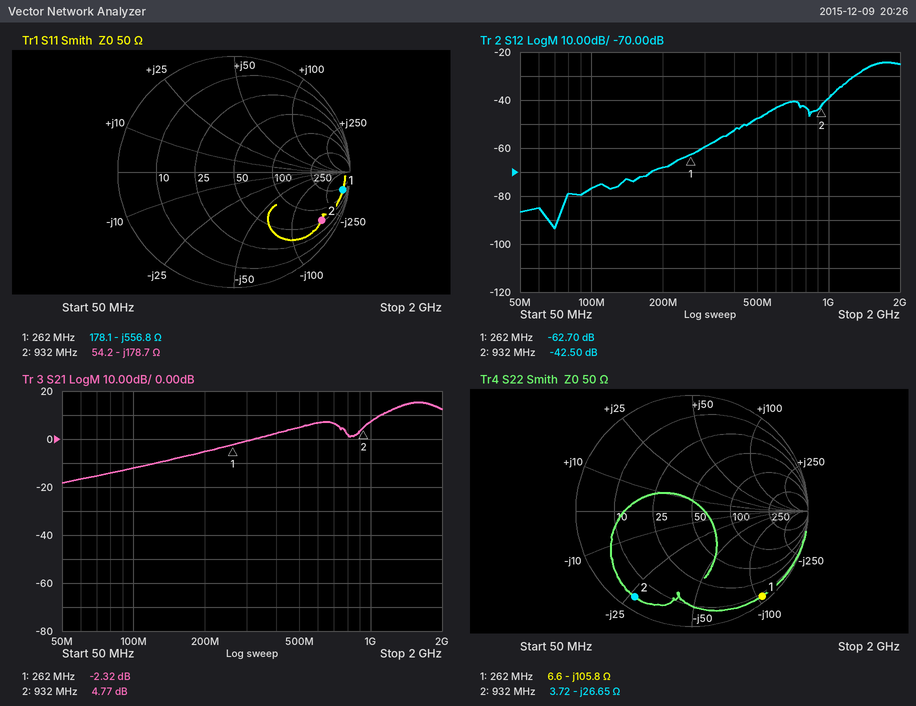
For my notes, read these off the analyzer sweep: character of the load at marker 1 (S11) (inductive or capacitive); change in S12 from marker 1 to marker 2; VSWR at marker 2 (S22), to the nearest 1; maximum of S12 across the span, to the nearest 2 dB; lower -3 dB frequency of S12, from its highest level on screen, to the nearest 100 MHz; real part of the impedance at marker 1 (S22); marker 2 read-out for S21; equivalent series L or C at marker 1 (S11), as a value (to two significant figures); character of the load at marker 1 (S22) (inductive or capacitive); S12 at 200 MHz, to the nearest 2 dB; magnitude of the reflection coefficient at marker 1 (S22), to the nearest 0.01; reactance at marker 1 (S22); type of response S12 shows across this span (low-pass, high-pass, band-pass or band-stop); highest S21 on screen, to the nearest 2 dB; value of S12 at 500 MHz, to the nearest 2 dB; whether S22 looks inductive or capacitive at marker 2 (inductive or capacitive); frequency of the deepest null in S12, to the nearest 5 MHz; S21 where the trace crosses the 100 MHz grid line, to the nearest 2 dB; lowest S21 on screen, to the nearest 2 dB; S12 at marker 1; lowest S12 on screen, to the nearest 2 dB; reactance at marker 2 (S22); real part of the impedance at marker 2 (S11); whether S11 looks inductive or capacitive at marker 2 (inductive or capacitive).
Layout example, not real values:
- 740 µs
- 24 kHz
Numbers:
- capacitive
- 20.20 dB
- 17
- -24 dB
- 1.4 GHz
- 6.6 Ω
- 4.77 dB
- 1.1 pF
- capacitive
- -68 dB
- 0.95
- -105.8 Ω
- high-pass
- 16 dB
- -48 dB
- capacitive
- 70 MHz
- -12 dB
- -18 dB
- -62.70 dB
- -94 dB
- -26.65 Ω
- 54.2 Ω
- capacitive
